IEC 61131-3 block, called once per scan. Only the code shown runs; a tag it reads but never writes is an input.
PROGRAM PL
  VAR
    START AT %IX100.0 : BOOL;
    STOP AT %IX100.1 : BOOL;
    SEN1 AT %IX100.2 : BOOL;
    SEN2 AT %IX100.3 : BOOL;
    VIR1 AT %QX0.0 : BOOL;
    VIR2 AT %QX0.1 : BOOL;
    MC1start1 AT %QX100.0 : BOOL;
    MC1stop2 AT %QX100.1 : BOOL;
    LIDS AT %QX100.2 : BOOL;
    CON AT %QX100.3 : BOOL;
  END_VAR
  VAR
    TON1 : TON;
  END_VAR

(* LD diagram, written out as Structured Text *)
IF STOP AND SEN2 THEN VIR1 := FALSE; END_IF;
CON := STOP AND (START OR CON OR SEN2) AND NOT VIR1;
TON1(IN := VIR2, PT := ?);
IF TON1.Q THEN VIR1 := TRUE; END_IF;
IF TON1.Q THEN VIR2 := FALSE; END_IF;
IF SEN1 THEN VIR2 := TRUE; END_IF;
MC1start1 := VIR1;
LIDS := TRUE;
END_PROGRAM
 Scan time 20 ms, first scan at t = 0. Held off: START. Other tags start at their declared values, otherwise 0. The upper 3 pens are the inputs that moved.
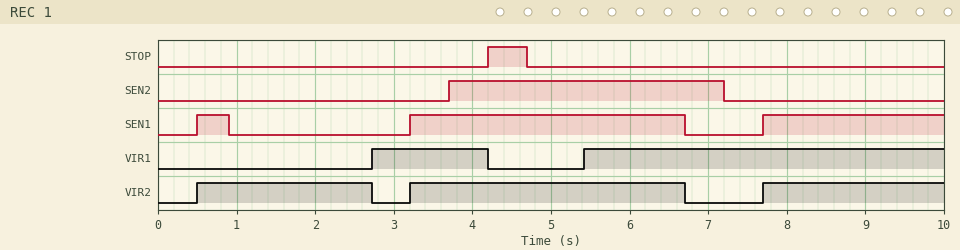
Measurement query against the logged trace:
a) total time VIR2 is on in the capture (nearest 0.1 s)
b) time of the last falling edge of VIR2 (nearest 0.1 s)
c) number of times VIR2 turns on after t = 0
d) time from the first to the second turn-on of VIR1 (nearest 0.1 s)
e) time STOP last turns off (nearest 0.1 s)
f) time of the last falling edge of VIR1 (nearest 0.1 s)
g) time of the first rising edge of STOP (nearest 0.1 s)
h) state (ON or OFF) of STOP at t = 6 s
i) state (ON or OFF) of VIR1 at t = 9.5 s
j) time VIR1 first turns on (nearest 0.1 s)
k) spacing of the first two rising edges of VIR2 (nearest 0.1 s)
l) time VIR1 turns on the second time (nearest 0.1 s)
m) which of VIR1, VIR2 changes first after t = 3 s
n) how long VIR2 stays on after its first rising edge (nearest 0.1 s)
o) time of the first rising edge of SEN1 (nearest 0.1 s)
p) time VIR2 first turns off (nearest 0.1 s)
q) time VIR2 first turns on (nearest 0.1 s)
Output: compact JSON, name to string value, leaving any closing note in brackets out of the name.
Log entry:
{"total time VIR2 is on in the capture": "8.0 s", "time of the last falling edge of VIR2": "6.7 s", "number of times VIR2 turns on after t = 0": "3", "time from the first to the second turn-on of VIR1": "2.7 s", "time STOP last turns off": "4.7 s", "time of the last falling edge of VIR1": "4.2 s", "time of the first rising edge of STOP": "4.2 s", "state (ON or OFF) of STOP at t = 6 s": "OFF", "state (ON or OFF) of VIR1 at t = 9.5 s": "ON", "time VIR1 first turns on": "2.7 s", "spacing of the first two rising edges of VIR2": "2.7 s", "time VIR1 turns on the second time": "5.4 s", "which of VIR1, VIR2 changes first after t = 3 s": "VIR2", "how long VIR2 stays on after its first rising edge": "2.2 s", "time of the first rising edge of SEN1": "0.5 s", "time VIR2 first turns off": "2.7 s", "time VIR2 first turns on": "0.5 s"}
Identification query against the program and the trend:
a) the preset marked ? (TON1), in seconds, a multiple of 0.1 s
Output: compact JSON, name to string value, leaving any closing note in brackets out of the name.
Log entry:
{"the preset marked ? (TON1), in seconds, a multiple of 0.1 s": "2.2 s"}
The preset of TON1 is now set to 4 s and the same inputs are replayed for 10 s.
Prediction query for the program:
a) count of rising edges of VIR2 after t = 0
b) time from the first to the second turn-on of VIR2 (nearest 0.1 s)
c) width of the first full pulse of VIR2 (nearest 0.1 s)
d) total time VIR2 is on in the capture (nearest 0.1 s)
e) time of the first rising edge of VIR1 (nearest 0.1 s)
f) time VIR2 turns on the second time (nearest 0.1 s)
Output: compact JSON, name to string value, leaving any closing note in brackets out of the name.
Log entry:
{"count of rising edges of VIR2 after t = 0": "2", "time from the first to the second turn-on of VIR2": "7.2 s", "width of the first full pulse of VIR2": "6.2 s", "total time VIR2 is on in the capture": "8.5 s", "time of the first rising edge of VIR1": "4.5 s", "time VIR2 turns on the second time": "7.7 s"}
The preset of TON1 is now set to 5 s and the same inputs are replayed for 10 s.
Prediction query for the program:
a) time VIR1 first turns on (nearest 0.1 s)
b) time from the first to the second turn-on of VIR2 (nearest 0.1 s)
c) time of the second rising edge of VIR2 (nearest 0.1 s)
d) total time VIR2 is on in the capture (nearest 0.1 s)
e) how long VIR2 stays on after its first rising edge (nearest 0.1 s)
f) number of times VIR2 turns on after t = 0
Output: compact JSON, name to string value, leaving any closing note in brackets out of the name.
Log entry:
{"time VIR1 first turns on": "5.5 s", "time from the first to the second turn-on of VIR2": "7.2 s", "time of the second rising edge of VIR2": "7.7 s", "total time VIR2 is on in the capture": "8.5 s", "how long VIR2 stays on after its first rising edge": "6.2 s", "number of times VIR2 turns on after t = 0": "2"}
